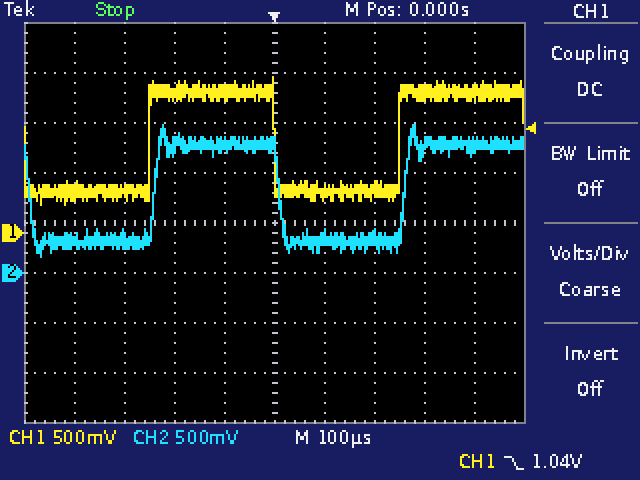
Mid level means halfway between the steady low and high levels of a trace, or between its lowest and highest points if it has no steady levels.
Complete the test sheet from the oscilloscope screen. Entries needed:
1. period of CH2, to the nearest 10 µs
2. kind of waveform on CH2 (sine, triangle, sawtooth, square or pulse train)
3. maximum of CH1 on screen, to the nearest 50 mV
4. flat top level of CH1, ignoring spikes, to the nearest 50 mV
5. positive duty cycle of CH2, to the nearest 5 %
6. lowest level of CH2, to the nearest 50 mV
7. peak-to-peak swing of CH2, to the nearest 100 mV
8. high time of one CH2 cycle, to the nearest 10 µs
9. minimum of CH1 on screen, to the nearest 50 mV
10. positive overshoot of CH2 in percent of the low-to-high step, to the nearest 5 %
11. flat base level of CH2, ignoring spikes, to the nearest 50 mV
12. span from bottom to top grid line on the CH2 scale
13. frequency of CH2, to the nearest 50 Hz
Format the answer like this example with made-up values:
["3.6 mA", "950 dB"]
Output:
["500 µs", "square", "1.55 V", "1.40 V", "50 %", "150 mV", "1.30 V", "250 µs", "300 mV", "20 %", "300 mV", "4 V", "2.00 kHz"]
